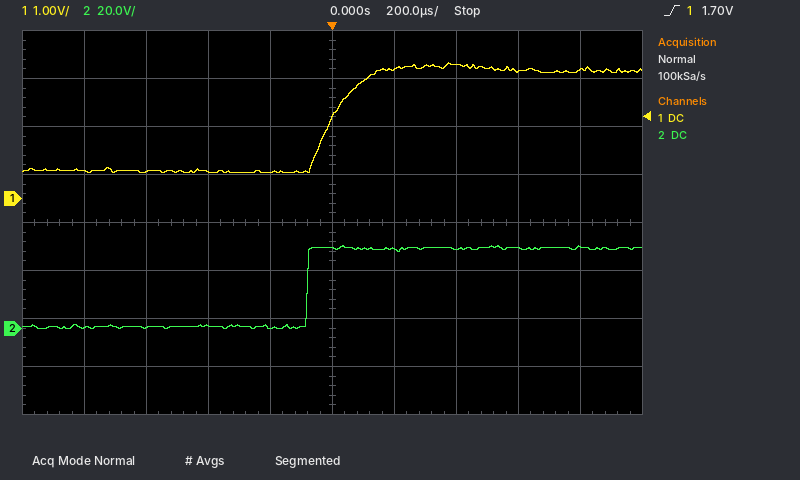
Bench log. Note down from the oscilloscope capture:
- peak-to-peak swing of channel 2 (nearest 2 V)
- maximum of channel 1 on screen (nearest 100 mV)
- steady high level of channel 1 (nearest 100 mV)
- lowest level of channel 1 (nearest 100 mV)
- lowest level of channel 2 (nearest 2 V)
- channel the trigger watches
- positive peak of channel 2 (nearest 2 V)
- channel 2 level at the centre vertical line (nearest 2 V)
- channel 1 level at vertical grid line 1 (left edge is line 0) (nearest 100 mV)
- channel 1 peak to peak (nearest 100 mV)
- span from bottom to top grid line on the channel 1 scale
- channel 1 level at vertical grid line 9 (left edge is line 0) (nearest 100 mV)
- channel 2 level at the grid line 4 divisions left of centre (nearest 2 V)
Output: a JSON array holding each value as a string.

["34 V", "2.8 V", "2.7 V", "500 mV", "0 V", "channel 1", "34 V", "34 V", "600 mV", "2.3 V", "8 V", "2.7 V", "0 V"]
